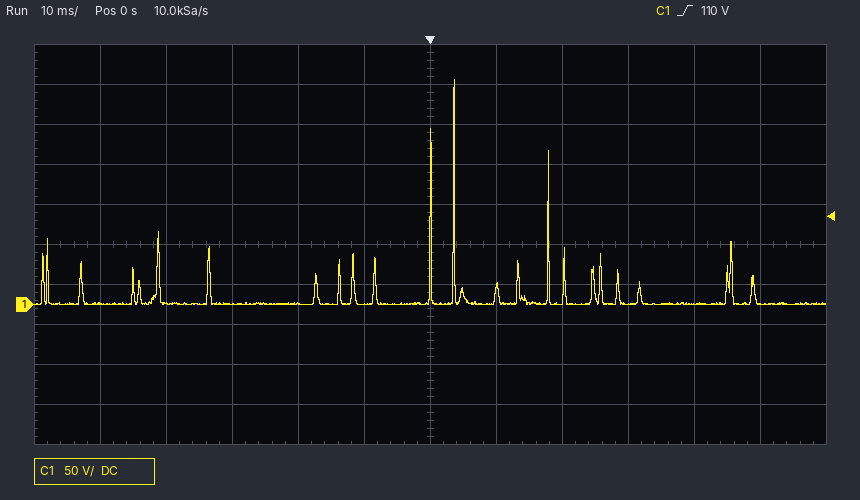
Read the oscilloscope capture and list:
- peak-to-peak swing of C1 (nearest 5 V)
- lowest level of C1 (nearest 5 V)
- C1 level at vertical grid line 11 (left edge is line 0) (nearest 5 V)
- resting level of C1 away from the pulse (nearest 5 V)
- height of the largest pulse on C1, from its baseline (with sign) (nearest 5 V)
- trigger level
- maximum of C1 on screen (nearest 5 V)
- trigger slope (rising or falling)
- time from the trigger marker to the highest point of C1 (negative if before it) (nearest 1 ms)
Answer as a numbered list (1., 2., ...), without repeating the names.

1. 280 V
2. 0 V
3. 0 V
4. 0 V
5. +280 V
6. 110 V
7. 280 V
8. rising
9. +4 ms
